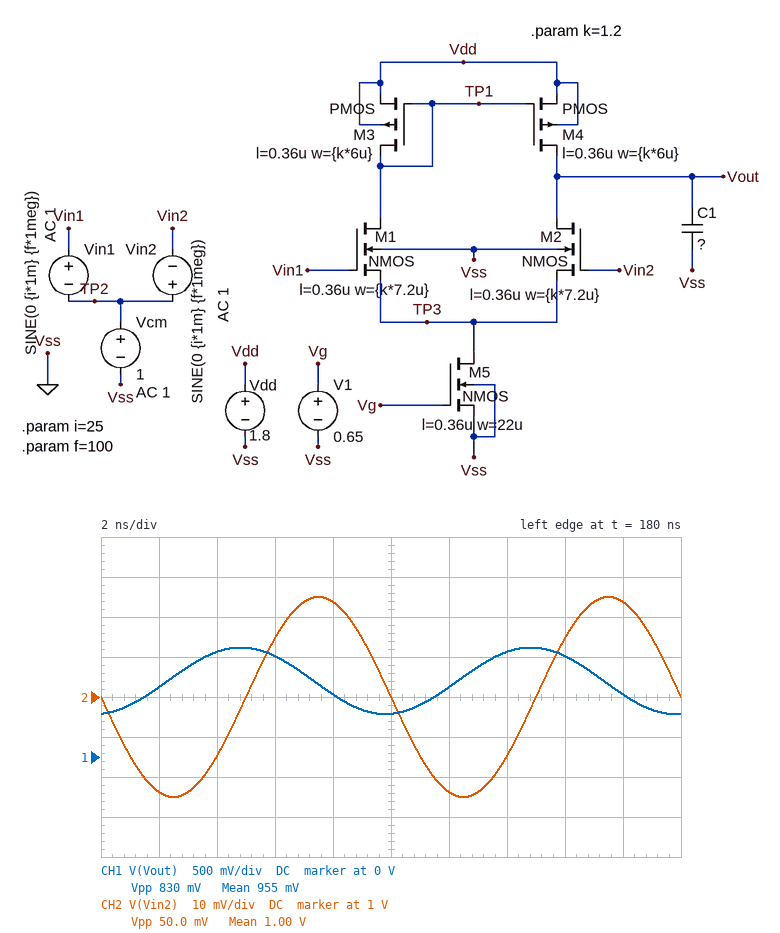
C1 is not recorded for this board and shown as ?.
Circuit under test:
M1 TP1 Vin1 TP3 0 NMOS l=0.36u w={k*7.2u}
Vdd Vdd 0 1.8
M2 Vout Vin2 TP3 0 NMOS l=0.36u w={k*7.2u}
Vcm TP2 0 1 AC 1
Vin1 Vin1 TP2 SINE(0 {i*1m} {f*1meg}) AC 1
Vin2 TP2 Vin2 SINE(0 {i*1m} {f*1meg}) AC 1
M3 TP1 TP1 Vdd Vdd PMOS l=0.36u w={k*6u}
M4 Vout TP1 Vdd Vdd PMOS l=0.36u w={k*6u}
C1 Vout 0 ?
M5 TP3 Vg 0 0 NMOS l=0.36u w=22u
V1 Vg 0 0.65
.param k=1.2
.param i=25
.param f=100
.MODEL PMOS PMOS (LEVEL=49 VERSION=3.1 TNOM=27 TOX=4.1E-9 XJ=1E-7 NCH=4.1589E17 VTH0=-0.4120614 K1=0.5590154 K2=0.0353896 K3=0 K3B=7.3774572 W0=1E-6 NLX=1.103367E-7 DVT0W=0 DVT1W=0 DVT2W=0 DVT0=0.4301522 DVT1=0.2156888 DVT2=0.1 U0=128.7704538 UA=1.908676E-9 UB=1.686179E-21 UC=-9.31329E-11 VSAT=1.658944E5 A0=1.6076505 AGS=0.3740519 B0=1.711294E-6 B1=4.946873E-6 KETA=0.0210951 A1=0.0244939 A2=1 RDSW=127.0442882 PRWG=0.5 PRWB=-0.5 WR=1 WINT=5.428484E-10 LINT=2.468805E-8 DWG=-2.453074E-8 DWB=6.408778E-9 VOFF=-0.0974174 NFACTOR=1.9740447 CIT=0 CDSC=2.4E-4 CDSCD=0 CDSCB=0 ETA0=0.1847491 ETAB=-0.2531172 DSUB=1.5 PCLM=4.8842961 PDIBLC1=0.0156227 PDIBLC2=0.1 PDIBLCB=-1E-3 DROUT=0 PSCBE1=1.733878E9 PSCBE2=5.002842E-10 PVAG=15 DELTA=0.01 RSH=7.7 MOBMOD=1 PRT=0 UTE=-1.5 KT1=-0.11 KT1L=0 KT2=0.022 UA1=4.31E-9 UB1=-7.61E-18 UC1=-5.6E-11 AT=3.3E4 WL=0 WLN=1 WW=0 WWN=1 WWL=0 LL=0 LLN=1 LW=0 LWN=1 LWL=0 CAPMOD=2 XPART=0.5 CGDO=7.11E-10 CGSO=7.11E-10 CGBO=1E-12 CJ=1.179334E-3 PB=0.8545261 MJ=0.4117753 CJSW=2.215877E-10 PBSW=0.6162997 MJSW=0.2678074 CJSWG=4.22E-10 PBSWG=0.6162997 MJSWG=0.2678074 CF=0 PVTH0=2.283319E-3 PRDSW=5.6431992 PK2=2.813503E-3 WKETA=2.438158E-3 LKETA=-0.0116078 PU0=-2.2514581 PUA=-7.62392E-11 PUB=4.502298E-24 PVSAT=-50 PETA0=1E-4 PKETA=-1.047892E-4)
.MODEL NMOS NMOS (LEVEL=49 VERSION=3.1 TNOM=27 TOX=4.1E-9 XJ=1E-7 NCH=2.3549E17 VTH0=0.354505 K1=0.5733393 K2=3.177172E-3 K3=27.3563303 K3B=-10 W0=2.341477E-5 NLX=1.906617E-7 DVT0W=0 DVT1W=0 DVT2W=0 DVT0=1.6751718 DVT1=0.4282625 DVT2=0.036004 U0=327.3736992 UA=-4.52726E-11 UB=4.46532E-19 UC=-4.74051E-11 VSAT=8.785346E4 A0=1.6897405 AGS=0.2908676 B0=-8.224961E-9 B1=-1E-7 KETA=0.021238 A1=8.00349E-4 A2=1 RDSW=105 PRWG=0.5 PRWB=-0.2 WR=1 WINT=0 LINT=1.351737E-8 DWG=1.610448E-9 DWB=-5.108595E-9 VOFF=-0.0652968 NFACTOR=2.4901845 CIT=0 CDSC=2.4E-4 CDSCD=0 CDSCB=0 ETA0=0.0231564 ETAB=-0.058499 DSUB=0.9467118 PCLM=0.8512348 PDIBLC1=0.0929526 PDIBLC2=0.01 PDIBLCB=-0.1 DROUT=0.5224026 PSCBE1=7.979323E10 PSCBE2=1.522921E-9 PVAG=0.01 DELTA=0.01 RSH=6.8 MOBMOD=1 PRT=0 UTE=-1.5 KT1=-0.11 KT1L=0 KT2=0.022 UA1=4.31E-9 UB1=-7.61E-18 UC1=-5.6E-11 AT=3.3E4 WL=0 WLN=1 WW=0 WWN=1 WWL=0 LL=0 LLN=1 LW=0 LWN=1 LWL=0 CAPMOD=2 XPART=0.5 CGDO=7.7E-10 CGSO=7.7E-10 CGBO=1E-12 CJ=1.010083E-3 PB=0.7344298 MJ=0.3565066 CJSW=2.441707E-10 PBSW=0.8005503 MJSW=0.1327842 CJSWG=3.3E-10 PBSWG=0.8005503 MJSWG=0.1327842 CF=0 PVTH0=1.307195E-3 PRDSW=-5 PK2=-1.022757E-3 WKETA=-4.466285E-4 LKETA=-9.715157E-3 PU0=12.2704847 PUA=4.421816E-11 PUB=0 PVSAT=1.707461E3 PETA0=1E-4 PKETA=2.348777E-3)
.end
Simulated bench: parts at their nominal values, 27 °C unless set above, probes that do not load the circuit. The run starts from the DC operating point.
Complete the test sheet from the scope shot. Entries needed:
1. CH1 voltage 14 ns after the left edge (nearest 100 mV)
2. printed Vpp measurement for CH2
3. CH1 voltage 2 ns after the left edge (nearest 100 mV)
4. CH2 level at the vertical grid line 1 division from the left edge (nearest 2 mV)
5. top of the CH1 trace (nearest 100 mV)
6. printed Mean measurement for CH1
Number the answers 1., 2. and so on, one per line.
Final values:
1. 1.3 V
2. 50.0 mV
3. 900 mV
4. 976 mV
5. 1.4 V
6. 955 mV
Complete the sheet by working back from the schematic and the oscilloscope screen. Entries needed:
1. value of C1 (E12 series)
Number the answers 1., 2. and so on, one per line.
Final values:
1. 180 fF
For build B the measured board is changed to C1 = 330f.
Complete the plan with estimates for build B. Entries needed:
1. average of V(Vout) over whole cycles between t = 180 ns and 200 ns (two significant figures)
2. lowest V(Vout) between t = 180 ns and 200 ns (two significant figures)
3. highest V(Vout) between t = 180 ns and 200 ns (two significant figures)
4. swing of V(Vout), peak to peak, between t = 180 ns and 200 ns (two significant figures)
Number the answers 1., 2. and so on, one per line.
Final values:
1. 940 mV
2. 700 mV
3. 1.2 V
4. 480 mV
